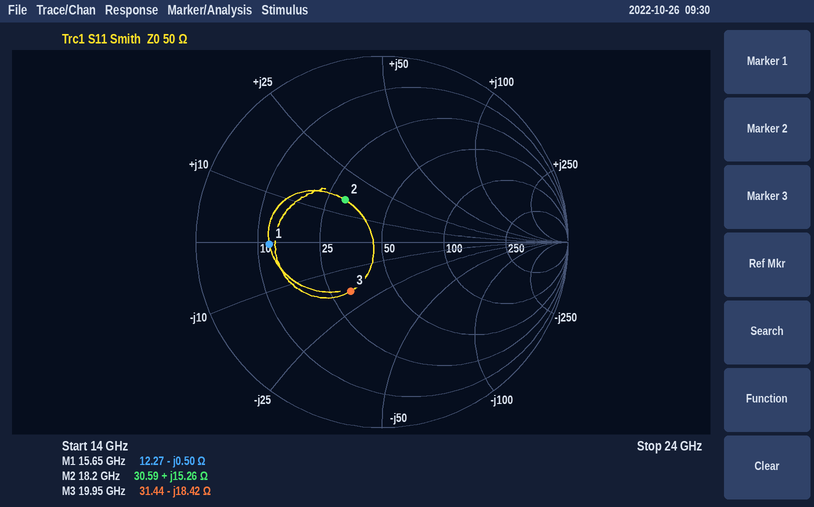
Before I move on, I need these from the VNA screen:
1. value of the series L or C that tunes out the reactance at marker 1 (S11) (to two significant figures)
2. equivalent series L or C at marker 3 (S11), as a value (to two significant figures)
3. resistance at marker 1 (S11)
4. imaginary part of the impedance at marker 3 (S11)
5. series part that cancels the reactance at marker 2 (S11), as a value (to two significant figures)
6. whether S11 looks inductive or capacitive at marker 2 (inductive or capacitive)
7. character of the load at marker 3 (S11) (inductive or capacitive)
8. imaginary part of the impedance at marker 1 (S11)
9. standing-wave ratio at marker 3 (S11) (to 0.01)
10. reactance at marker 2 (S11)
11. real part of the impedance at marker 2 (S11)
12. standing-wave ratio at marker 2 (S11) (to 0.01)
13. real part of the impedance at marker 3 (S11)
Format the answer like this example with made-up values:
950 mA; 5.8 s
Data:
5.1 pH; 430 fF; 12.27 Ω; -18.42 Ω; 570 fF; inductive; capacitive; -0.50 Ω; 1.91; +15.26 Ω; 30.59 Ω; 1.86; 31.44 Ω
